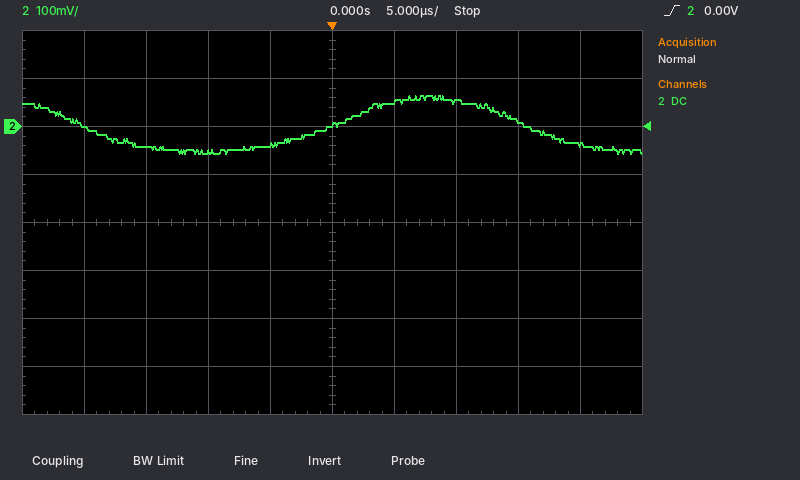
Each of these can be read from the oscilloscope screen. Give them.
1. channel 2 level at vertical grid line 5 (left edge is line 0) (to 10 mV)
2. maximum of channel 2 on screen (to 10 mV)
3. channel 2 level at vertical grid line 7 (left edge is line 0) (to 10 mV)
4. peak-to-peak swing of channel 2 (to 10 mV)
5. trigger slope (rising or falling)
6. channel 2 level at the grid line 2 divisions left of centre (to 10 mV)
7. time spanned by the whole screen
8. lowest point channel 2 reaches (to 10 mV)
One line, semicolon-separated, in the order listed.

0 mV; 60 mV; 50 mV; 120 mV; rising; -50 mV; 50 µs; -60 mV
